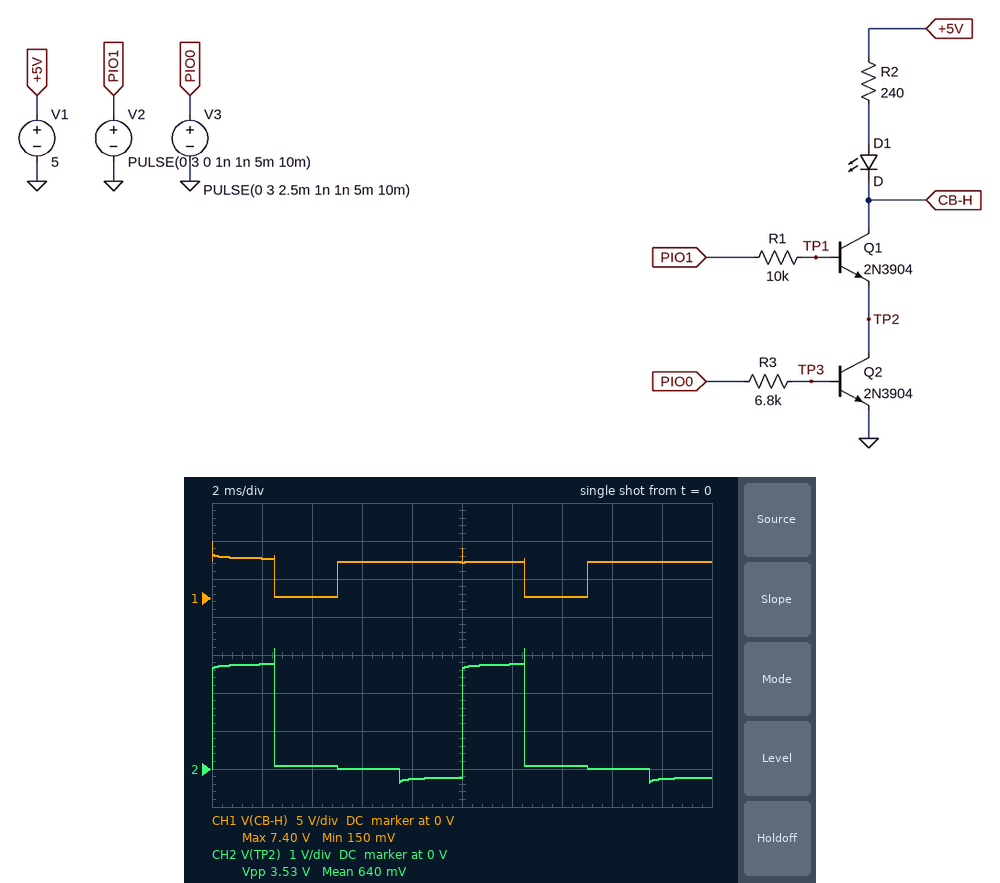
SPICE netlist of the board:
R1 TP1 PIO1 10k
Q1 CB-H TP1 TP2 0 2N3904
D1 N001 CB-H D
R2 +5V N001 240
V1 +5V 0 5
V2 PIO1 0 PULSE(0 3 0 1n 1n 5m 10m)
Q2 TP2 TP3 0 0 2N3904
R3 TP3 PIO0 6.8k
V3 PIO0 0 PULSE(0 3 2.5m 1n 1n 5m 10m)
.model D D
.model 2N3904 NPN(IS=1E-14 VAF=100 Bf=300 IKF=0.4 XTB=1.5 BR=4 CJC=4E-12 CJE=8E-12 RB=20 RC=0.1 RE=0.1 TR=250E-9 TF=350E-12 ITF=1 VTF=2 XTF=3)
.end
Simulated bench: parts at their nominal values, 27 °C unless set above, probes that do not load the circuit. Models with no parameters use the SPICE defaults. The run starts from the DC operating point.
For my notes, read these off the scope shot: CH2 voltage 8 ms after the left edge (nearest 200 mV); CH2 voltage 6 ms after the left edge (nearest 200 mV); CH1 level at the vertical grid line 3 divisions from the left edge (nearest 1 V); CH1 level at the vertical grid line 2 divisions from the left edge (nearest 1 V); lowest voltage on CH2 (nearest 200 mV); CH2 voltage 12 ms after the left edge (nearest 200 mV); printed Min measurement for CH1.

-200 mV
0 V
5 V
0 V
-400 mV
2.8 V
150 mV
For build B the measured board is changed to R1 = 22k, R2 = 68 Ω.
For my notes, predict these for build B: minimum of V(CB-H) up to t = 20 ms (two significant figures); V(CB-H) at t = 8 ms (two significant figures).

2.4 V
4.7 V
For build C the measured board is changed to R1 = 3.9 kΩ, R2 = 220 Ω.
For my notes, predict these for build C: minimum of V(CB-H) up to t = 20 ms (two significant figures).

150 mV
